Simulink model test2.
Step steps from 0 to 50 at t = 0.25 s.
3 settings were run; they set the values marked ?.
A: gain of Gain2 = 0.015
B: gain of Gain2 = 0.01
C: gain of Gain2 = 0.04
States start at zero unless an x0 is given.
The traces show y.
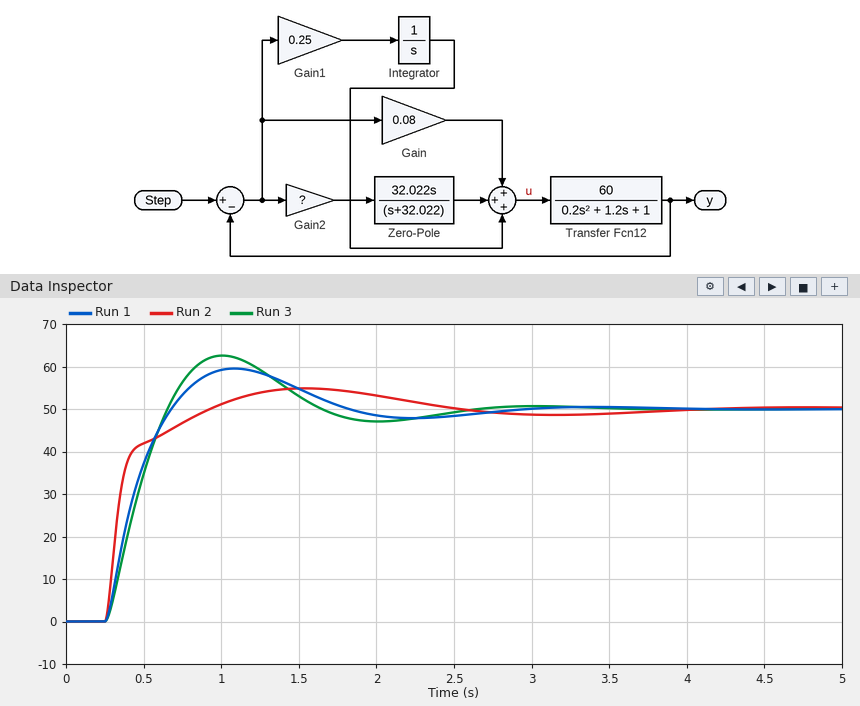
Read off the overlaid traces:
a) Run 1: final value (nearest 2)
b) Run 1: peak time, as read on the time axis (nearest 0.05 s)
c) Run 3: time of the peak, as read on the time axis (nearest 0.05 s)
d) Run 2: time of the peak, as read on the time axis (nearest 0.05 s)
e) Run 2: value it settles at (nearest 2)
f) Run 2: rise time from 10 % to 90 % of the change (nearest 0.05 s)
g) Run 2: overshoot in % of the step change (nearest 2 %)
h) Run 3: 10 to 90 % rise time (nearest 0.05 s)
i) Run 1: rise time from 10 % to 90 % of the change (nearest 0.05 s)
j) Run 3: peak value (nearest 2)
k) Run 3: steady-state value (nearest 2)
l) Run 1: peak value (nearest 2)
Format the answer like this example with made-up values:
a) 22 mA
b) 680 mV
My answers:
a) 50
b) 1.10 s
c) 1.00 s
d) 1.55 s
e) 50
f) 0.40 s
g) 10 %
h) 0.30 s
i) 0.30 s
j) 62
k) 50
l) 60
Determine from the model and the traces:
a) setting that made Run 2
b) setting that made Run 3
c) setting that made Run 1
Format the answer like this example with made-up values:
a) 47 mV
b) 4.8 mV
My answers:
a) C
b) B
c) A
